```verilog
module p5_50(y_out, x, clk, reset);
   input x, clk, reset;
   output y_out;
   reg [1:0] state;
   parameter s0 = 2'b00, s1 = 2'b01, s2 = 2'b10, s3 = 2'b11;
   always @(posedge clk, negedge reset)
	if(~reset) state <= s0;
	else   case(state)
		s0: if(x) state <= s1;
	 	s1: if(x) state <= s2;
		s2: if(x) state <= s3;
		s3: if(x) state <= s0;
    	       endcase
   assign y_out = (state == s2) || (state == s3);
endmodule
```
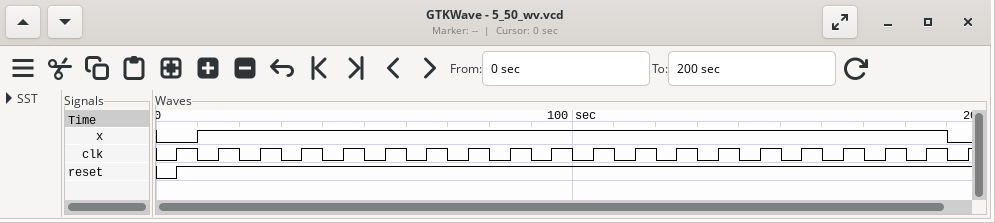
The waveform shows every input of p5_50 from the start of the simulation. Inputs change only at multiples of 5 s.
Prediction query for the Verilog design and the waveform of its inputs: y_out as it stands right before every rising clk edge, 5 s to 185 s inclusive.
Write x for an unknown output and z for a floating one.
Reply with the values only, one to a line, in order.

0 0 0 1 1 0 0 1 1 0 0 1 1 0 0 1 1 0 0
